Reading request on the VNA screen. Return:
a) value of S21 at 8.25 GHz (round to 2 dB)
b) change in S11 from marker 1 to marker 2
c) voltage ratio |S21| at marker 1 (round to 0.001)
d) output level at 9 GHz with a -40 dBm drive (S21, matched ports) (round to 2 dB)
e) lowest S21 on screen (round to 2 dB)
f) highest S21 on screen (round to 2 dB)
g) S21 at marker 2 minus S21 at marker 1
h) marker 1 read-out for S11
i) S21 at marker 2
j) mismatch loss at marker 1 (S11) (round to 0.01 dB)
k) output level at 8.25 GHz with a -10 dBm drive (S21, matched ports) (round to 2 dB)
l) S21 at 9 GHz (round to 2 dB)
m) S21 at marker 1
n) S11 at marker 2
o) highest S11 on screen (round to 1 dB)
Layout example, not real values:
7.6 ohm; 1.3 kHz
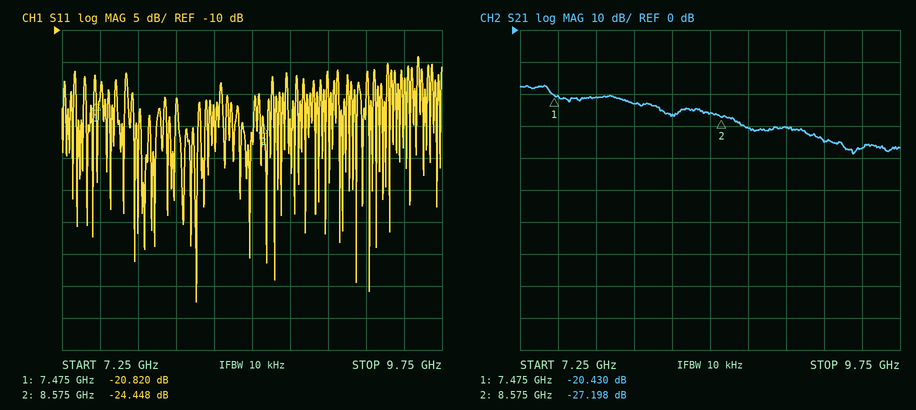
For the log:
-26 dB; -3.628 dB; 0.095; -70 dBm; -38 dB; -18 dB; -6.768 dB; -20.820 dB; -27.198 dB; 0.04 dB; -36 dBm; -30 dB; -20.430 dB; -24.448 dB; -14 dB
